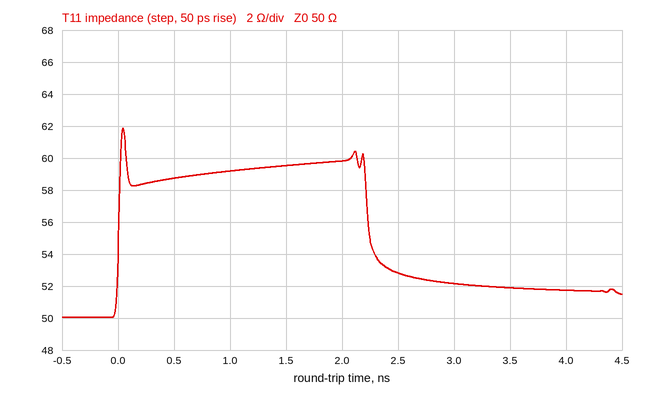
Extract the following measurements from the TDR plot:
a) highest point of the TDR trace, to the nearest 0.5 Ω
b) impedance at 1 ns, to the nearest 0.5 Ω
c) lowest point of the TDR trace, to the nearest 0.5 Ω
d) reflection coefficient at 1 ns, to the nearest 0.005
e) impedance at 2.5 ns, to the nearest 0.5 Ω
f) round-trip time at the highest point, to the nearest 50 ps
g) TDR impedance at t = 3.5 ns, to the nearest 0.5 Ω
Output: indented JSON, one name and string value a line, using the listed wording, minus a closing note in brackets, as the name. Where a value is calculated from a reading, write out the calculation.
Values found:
{
  "highest point of the TDR trace, to the nearest 0.5 Ω": "62.0 Ω",
  "impedance at 1 ns, to the nearest 0.5 Ω": "59.0 Ω",
  "lowest point of the TDR trace, to the nearest 0.5 Ω": "50.0 Ω",
  "reflection coefficient at 1 ns, to the nearest 0.005": "(59 − 50)/(59 + 50) ≈ +0.0826, so +0.085 to the nearest 0.005",
  "impedance at 2.5 ns, to the nearest 0.5 Ω": "53.0 Ω",
  "round-trip time at the highest point, to the nearest 50 ps": "50 ps",
  "TDR impedance at t = 3.5 ns, to the nearest 0.5 Ω": "52.0 Ω"
}
